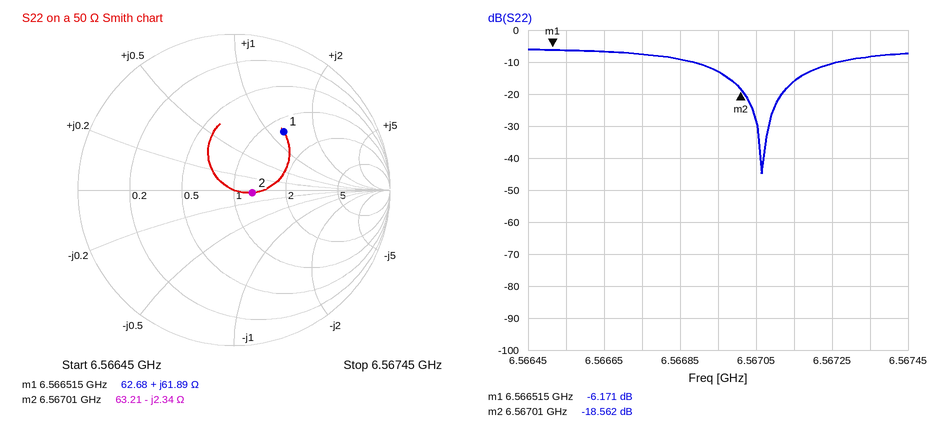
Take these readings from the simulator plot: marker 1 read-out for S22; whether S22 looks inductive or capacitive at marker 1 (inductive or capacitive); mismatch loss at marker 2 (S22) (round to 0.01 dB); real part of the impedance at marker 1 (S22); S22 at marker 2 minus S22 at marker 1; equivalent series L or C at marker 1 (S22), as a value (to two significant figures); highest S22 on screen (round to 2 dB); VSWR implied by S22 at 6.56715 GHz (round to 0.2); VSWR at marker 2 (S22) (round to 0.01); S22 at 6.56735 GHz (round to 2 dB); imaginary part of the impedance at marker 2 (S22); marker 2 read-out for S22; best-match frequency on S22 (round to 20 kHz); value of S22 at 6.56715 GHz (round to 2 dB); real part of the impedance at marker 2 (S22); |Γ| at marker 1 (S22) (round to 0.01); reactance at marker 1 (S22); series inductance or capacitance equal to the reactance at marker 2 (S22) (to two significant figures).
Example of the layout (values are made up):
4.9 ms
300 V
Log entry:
-6.171 dB
inductive
0.06 dB
62.68 Ω
-12.391 dB
1.5 nH
-6 dB
1.4
1.27
-8 dB
-2.34 Ω
-18.562 dB
6.56706 GHz
-16 dB
63.21 Ω
0.49
+61.89 Ω
10 pF
